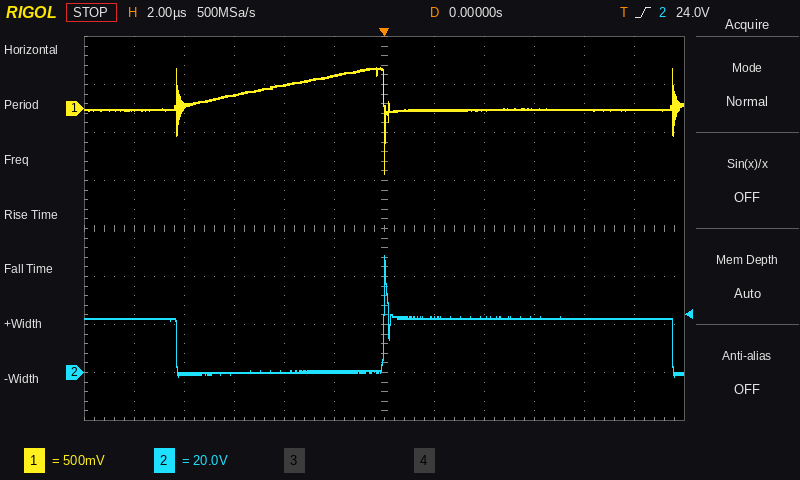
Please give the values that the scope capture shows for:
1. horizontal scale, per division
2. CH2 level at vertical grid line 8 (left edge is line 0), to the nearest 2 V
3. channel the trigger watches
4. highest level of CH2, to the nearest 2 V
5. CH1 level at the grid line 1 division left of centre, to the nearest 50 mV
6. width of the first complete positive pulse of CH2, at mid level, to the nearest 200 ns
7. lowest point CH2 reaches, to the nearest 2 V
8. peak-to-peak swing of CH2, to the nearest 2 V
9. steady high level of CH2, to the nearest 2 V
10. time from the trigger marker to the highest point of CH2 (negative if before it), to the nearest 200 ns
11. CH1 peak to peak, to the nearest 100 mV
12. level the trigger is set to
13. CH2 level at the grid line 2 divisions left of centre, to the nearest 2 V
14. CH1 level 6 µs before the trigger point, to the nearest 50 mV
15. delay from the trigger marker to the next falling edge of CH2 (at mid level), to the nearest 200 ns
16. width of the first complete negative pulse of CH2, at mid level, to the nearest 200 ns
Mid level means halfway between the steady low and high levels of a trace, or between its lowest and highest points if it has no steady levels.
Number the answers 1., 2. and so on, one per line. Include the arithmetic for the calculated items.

1. 2 µs
2. 22 V
3. CH2
4. 48 V
5. 350 mV
6. 11.6 µs
7. -2 V
8. 48 V − (-2 V) = 50 V
9. 22 V
10. 0.0 µs
11. 1.10 V
12. 24.0 V
13. 0 V
14. 150 mV
15. 11.6 µs
16. 8.2 µs
